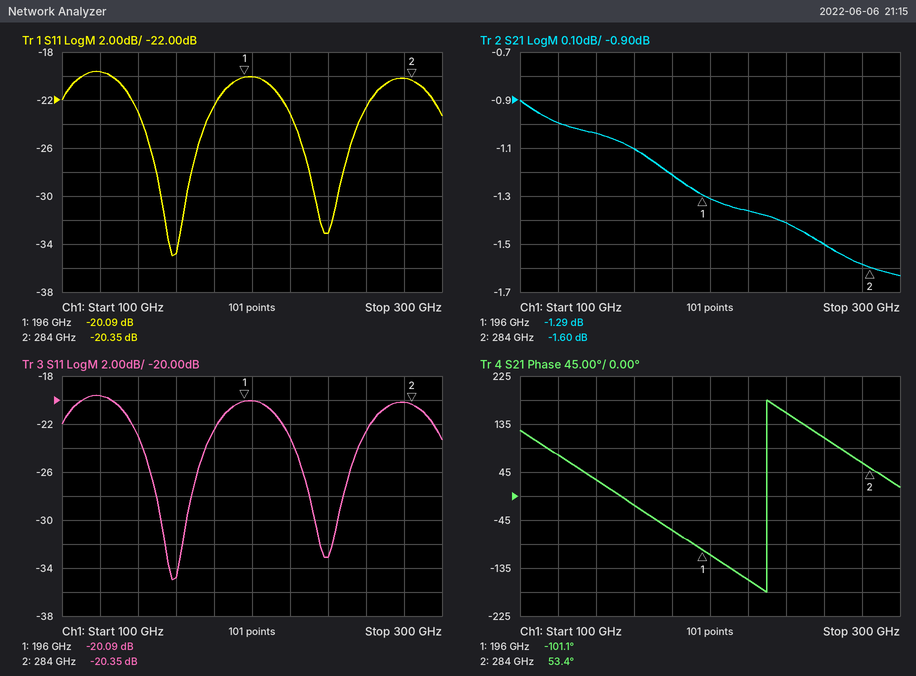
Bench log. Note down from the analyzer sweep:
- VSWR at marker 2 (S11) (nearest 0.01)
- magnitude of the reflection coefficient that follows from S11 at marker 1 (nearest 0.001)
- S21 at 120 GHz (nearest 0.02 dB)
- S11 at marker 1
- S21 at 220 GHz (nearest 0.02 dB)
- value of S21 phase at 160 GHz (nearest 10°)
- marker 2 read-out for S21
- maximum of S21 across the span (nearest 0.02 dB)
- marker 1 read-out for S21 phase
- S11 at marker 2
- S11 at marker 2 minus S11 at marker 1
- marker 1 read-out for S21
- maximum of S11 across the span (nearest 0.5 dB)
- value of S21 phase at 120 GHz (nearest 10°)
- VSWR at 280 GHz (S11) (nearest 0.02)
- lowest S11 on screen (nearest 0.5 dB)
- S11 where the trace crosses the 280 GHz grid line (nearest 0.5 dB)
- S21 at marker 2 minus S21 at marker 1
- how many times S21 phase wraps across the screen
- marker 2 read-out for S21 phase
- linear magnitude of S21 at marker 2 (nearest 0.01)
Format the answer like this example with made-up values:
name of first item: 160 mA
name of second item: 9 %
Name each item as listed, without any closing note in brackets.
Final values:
VSWR at marker 2 (S11): 1.21
magnitude of the reflection coefficient that follows from S11 at marker 1: 0.099
S21 at 120 GHz: -1.00 dB
S11 at marker 1: -20.09 dB
S21 at 220 GHz: -1.36 dB
value of S21 phase at 160 GHz: -20°
marker 2 read-out for S21: -1.60 dB
maximum of S21 across the span: -0.90 dB
marker 1 read-out for S21 phase: -101.1°
S11 at marker 2: -20.35 dB
S11 at marker 2 minus S11 at marker 1: -0.26 dB
marker 1 read-out for S21: -1.29 dB
maximum of S11 across the span: -19.5 dB
value of S21 phase at 120 GHz: 80°
VSWR at 280 GHz (S11): 1.22
lowest S11 on screen: -35.0 dB
S11 where the trace crosses the 280 GHz grid line: -20.0 dB
S21 at marker 2 minus S21 at marker 1: -0.31 dB
how many times S21 phase wraps across the screen: 1
marker 2 read-out for S21 phase: 53.4°
linear magnitude of S21 at marker 2: 0.83
